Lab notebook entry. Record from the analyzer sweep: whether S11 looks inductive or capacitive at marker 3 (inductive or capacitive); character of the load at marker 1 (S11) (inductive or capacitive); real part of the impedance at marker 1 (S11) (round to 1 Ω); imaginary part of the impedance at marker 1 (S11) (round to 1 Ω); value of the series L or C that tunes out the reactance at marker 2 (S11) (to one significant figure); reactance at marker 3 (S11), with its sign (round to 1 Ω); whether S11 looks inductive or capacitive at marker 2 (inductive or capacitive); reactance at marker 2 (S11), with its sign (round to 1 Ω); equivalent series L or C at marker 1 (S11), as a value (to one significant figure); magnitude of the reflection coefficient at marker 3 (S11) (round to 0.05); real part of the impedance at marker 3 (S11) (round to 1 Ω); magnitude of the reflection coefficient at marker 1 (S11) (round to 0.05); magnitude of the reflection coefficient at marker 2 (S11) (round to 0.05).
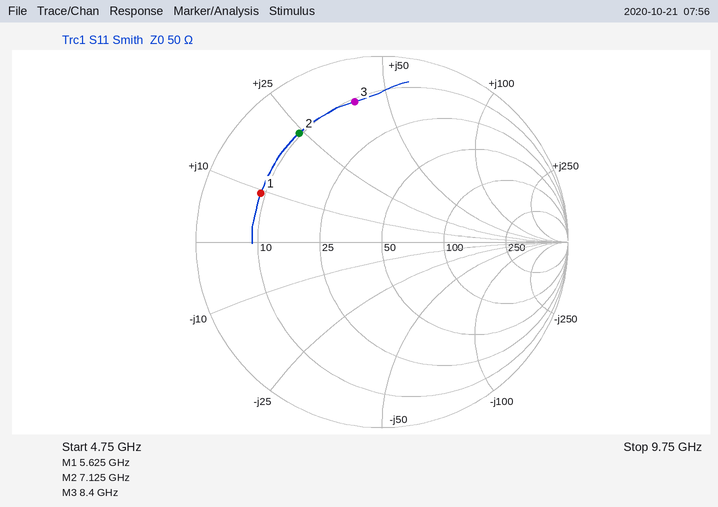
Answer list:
inductive
inductive
9 Ω
+9 Ω
900 fF
+40 Ω
inductive
+24 Ω
300 pH
0.75
11 Ω
0.70
0.75
